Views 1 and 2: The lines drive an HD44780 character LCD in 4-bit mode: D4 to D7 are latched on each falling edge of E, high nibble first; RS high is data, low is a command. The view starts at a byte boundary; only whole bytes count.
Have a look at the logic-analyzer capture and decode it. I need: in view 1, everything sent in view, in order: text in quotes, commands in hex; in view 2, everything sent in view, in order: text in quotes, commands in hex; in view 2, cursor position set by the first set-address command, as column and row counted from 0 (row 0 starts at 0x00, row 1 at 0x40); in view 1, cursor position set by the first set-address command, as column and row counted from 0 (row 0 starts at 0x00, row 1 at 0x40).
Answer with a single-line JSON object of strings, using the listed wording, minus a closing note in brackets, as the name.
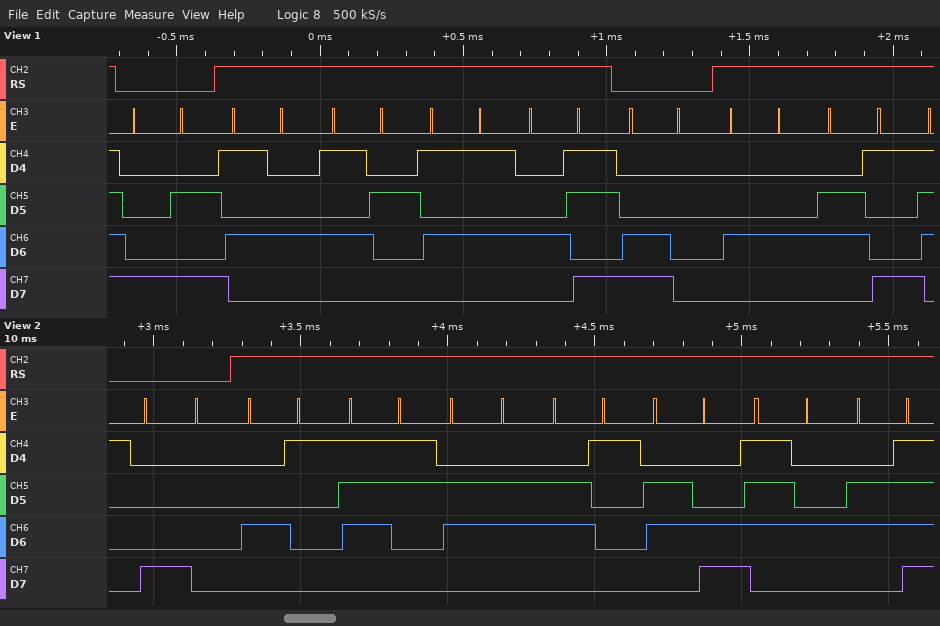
{"in view 1, everything sent in view, in order: text in quotes, commands in hex": "0x8A \"TRUK\" 0xC0 \"Di\"", "in view 2, everything sent in view, in order: text in quotes, commands in hex": "0x80 \"Asfalto\"", "in view 2, cursor position set by the first set-address command, as column and row counted from 0": "column 0, row 0", "in view 1, cursor position set by the first set-address command, as column and row counted from 0": "column 10, row 0"}
